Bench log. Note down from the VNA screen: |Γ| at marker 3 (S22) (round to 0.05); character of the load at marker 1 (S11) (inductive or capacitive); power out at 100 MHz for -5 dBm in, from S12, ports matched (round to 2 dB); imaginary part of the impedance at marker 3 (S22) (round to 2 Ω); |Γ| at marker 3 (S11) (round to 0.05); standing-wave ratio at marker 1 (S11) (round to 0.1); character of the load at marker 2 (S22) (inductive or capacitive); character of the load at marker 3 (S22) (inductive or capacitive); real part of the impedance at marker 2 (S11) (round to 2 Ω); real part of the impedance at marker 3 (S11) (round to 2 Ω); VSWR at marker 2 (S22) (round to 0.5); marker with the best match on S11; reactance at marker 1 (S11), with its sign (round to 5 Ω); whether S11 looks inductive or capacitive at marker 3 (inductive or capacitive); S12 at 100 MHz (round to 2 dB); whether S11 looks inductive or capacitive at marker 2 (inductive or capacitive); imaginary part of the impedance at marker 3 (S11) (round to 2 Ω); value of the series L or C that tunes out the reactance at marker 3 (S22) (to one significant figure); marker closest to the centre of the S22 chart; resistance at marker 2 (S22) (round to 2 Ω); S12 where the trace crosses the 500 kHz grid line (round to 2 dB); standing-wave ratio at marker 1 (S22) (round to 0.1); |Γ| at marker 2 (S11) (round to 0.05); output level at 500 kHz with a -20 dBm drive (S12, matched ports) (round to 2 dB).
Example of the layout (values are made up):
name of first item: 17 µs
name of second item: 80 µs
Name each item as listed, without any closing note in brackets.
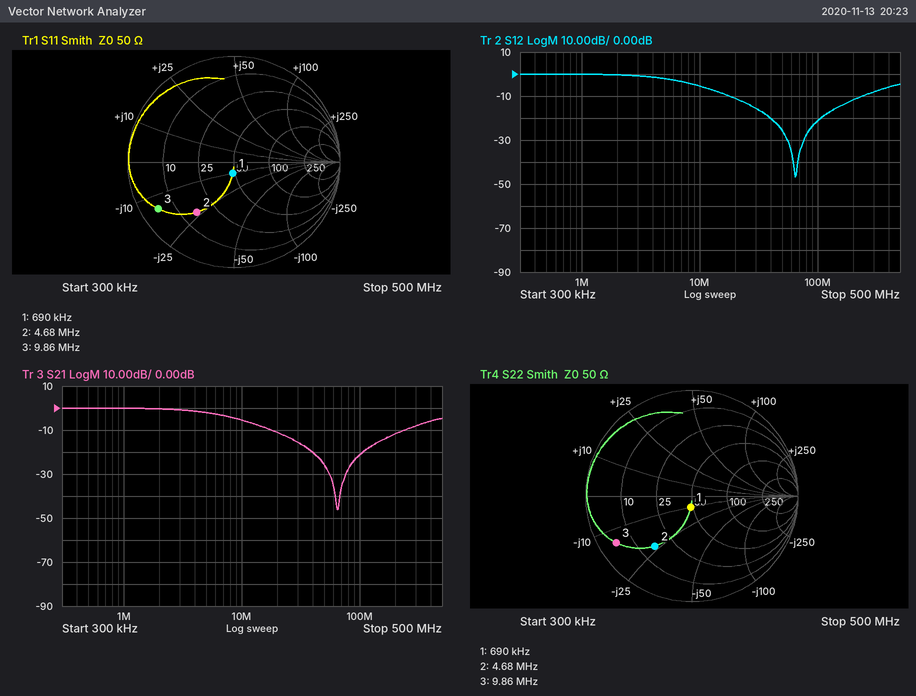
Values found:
|Γ| at marker 3 (S22): 0.85
character of the load at marker 1 (S11): capacitive
power out at 100 MHz for -5 dBm in, from S12, ports matched: -26 dBm
imaginary part of the impedance at marker 3 (S22): -14 Ω
|Γ| at marker 3 (S11): 0.85
standing-wave ratio at marker 1 (S11): 1.2
character of the load at marker 2 (S22): capacitive
character of the load at marker 3 (S22): capacitive
real part of the impedance at marker 2 (S11): 16 Ω
real part of the impedance at marker 3 (S11): 4 Ω
VSWR at marker 2 (S22): 4.0
marker with the best match on S11: marker 1
reactance at marker 1 (S11), with its sign: -10 Ω
whether S11 looks inductive or capacitive at marker 3: capacitive
S12 at 100 MHz: -22 dB
whether S11 looks inductive or capacitive at marker 2: capacitive
imaginary part of the impedance at marker 3 (S11): -14 Ω
value of the series L or C that tunes out the reactance at marker 3 (S22): 200 nH
marker closest to the centre of the S22 chart: marker 1
resistance at marker 2 (S22): 16 Ω
S12 where the trace crosses the 500 kHz grid line: 0 dB
standing-wave ratio at marker 1 (S22): 1.2
|Γ| at marker 2 (S11): 0.60
output level at 500 kHz with a -20 dBm drive (S12, matched ports): -20 dBm
